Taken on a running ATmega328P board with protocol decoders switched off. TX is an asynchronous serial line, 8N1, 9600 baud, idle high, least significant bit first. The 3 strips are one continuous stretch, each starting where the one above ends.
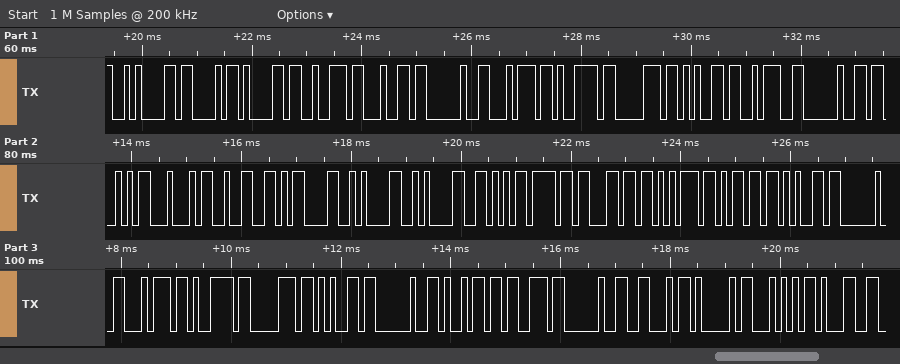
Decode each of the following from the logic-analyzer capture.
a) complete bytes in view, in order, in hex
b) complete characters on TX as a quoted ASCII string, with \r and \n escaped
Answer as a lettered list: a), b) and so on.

a) 0x0A 0x43 0x61 0x72 0x64 0x20 0x74 0x79 0x70 0x65 0x3A 0x20 0x53 0x44 0x32 0x0D 0x0A 0x0A 0x56 0x6F 0x6C 0x75 0x6D 0x65 0x20 0x74 0x79 0x70 0x65 0x20 0x69 0x73 0x20 0x46 0x41 0x54 0x31
b) "\nCard type: SD2\r\n\nVolume type is FAT1"
